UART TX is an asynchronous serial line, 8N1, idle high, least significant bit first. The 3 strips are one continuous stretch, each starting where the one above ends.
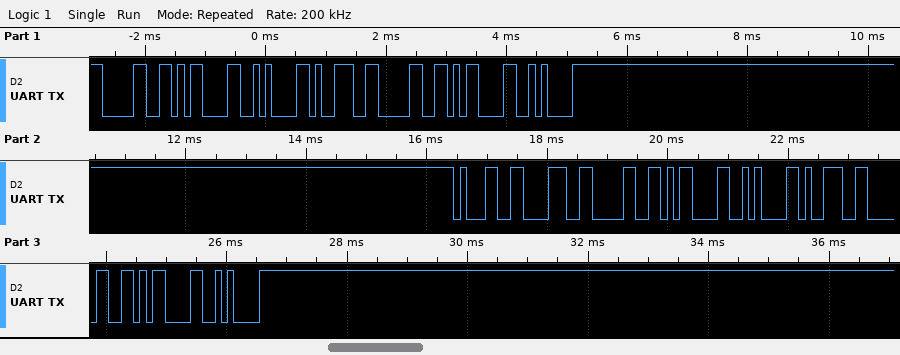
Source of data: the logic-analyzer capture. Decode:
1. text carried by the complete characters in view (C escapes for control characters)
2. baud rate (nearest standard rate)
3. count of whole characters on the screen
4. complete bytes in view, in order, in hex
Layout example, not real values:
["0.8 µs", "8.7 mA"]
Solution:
["\"0\\r\\n90\\r\\n180\\r\\n90\\r\\n\"", "9600 baud", "16", "30 0D 0A 39 30 0D 0A 31 38 30 0D 0A 39 30 0D 0A"]
